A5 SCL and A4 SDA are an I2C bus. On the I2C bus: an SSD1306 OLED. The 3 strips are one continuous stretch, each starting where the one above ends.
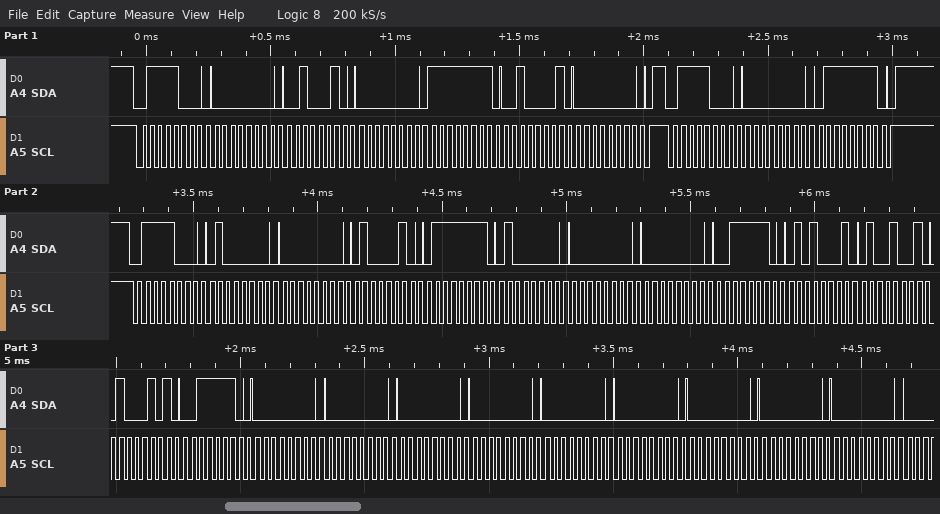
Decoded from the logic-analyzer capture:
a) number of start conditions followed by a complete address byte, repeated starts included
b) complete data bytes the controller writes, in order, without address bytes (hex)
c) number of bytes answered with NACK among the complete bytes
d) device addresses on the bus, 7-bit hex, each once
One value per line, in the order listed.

3
00 22 00 FF 21 00 00 7F 40 00 42 7F 40 00 00 3E 51 49 45 3E 00 00 00 00 00 00 00 00 00
0
0x3C
